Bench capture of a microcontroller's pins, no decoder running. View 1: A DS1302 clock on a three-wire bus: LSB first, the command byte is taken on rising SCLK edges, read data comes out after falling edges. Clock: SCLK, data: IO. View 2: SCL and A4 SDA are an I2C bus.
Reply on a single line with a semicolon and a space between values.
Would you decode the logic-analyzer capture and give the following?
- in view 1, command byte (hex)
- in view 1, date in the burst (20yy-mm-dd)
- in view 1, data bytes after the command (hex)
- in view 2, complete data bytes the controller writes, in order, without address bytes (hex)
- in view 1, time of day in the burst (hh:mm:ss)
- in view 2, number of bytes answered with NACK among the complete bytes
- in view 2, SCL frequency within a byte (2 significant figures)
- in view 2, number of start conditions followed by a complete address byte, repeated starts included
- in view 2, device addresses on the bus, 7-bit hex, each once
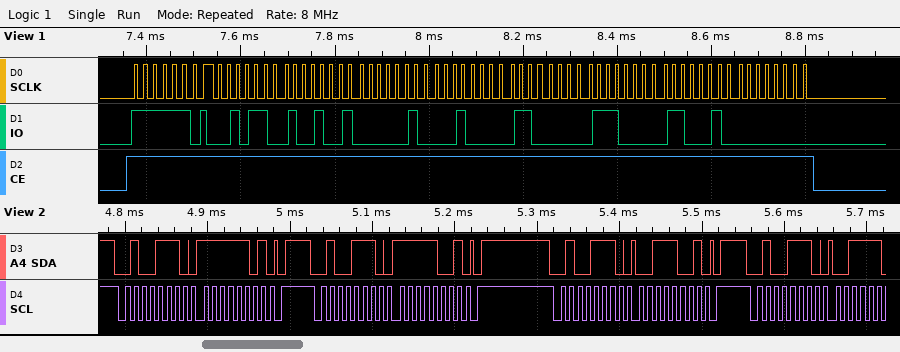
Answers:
0xBF; 2023-03-04; 34 49 20 04 03 07 23 00; FD F9 39; 20:49:34; 0; 100 kHz; 4; 0x27
